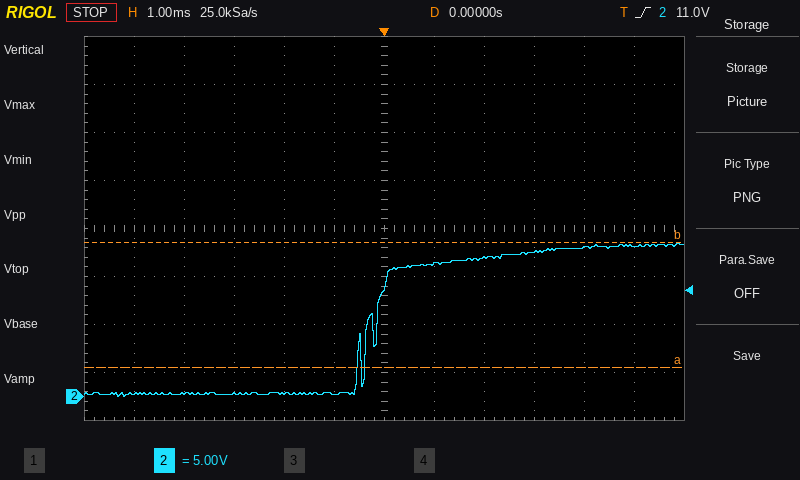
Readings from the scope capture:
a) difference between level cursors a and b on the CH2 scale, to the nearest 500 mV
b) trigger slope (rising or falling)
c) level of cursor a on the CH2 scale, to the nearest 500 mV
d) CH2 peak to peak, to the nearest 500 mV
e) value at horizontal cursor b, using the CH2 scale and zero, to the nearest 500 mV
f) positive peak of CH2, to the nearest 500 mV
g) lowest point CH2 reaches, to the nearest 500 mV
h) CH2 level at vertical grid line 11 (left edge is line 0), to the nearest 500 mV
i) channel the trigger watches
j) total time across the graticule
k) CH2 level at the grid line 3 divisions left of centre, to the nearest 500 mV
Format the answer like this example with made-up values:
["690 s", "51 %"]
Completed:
["13.0 V", "rising", "3.0 V", "16.0 V", "16.0 V", "16.0 V", "0.0 V", "15.5 V", "CH2", "12 ms", "500 mV"]
